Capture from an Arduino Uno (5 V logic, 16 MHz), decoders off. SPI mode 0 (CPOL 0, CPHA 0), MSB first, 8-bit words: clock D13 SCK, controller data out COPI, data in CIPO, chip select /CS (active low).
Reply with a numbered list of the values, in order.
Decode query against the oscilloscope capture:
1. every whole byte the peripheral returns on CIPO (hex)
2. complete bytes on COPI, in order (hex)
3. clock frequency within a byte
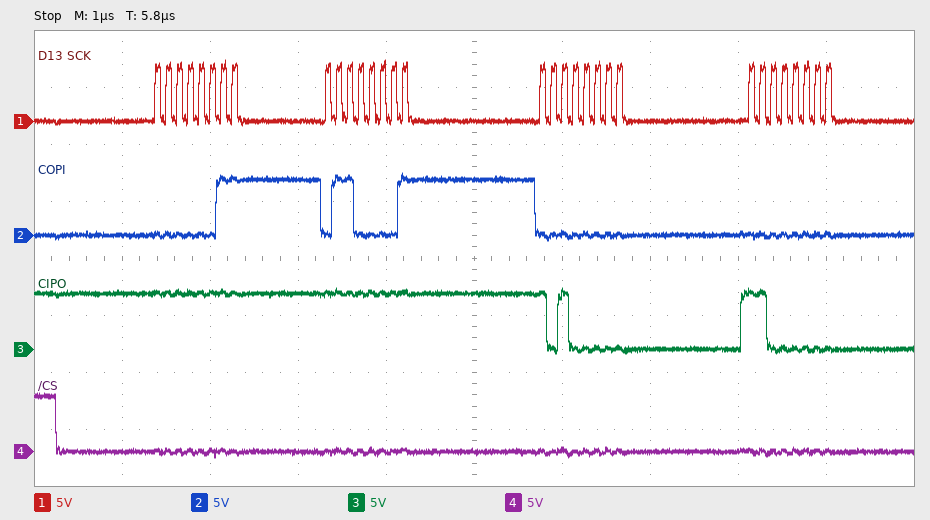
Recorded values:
1. FF FF A0 C0
2. 03 61 00 00
3. 8 MHz
